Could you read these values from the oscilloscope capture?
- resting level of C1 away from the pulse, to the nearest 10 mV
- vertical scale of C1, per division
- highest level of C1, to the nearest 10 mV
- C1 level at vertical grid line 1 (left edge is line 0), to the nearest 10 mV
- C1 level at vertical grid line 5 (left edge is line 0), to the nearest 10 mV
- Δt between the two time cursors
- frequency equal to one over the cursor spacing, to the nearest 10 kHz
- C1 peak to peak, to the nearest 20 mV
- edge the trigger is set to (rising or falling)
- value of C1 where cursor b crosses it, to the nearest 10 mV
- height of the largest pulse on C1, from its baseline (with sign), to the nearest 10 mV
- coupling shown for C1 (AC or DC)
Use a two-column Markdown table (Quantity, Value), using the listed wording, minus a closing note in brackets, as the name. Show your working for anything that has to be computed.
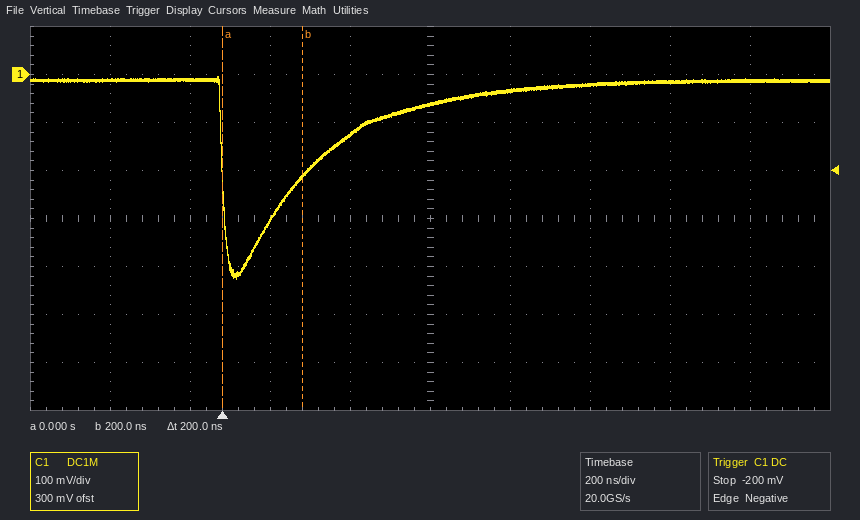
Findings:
| Quantity | Value |
|---|---|
| resting level of C1 away from the pulse, to the nearest 10 mV | -10 mV |
| vertical scale of C1, per division | 100 mV |
| highest level of C1, to the nearest 10 mV | 0 mV |
| C1 level at vertical grid line 1 (left edge is line 0), to the nearest 10 mV | -10 mV |
| C1 level at vertical grid line 5 (left edge is line 0), to the nearest 10 mV | -60 mV |
| Δt between the two time cursors | 200 ns |
| frequency equal to one over the cursor spacing, to the nearest 10 kHz | 1 / 200 ns ≈ 5.00 MHz |
| C1 peak to peak, to the nearest 20 mV | 420 mV |
| edge the trigger is set to | falling |
| value of C1 where cursor b crosses it, to the nearest 10 mV | -210 mV |
| height of the largest pulse on C1, from its baseline (with sign), to the nearest 10 mV | -410 mV |
| coupling shown for C1 | DC |
